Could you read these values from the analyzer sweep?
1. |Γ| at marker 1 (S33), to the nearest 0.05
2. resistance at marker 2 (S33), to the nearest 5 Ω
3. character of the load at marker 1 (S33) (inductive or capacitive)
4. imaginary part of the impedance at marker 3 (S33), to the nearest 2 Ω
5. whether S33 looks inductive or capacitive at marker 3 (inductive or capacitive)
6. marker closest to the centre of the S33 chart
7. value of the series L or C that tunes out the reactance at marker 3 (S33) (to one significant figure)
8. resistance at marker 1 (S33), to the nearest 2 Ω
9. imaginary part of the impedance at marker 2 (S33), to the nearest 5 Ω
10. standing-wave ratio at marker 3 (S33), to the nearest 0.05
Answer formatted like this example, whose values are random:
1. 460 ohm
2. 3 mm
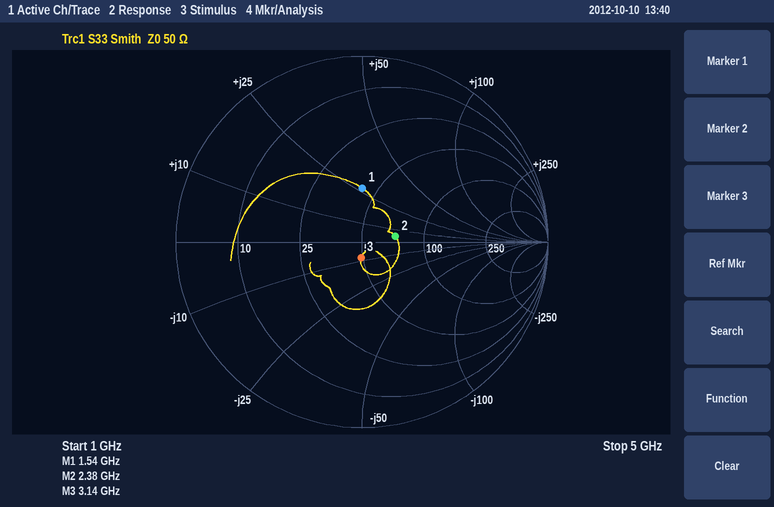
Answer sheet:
1. 0.30
2. 70 Ω
3. inductive
4. -8 Ω
5. capacitive
6. marker 3
7. 400 pH
8. 42 Ω
9. +5 Ω
10. 1.20
